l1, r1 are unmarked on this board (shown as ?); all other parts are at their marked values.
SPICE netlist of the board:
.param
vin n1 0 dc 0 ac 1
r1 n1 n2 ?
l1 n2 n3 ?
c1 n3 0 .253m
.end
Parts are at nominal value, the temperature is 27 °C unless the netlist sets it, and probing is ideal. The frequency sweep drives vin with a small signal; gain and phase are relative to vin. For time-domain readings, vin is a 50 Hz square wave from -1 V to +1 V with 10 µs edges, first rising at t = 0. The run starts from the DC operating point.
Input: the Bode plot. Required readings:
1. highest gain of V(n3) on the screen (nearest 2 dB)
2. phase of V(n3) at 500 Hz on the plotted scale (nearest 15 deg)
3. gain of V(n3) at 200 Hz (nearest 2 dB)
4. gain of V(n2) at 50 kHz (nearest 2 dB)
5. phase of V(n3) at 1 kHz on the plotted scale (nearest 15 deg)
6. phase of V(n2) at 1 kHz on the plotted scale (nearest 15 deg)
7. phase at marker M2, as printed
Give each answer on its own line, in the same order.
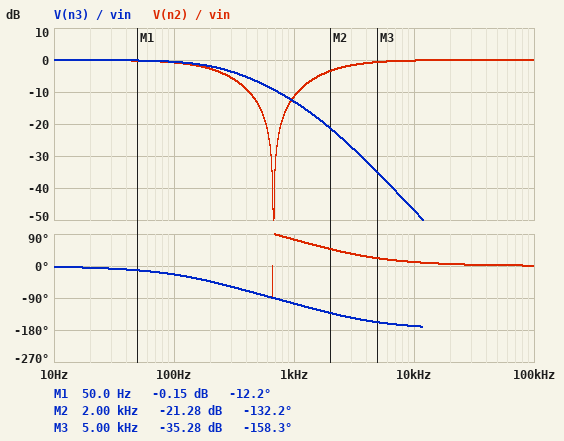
0 dB
-75 deg
-2 dB
0 dB
-105 deg
75 deg
-132.2 deg
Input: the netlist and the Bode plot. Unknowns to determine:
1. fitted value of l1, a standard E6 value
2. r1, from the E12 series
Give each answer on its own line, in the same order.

220 µH
2.7 Ω
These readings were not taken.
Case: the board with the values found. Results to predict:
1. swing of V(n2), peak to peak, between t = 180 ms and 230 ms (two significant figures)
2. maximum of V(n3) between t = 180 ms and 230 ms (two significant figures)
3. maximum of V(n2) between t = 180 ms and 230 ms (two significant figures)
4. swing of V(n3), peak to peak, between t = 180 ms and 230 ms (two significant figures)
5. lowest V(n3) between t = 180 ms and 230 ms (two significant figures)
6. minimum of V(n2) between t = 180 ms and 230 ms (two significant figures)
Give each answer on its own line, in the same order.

2.0 V
1.0 V
1.0 V
2.0 V
-1.0 V
-1.0 V
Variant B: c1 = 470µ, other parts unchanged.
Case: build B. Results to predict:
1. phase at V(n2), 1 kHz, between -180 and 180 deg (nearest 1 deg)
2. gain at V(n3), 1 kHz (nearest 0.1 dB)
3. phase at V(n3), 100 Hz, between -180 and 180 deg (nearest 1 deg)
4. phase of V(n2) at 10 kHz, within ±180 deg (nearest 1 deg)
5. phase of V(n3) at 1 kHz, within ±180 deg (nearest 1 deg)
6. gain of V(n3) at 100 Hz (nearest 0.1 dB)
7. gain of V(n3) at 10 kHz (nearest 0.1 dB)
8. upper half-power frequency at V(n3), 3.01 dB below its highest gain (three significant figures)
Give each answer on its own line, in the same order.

69 deg
-18.6 dB
-40 deg
11 deg
-111 deg
-1.9 dB
-52.4 dB
134 Hz
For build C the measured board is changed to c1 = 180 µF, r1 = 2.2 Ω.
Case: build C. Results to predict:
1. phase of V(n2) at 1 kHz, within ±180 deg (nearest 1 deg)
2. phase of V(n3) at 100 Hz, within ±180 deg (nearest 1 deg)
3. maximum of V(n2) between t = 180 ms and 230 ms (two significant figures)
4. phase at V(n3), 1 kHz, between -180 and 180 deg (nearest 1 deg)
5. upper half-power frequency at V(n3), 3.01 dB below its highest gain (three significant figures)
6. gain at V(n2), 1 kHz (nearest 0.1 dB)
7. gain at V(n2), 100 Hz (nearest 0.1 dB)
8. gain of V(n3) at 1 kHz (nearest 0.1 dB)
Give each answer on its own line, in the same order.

77 deg
-14 deg
1.0 V
-103 deg
518 Hz
-13.1 dB
-0.3 dB
-8.1 dB
